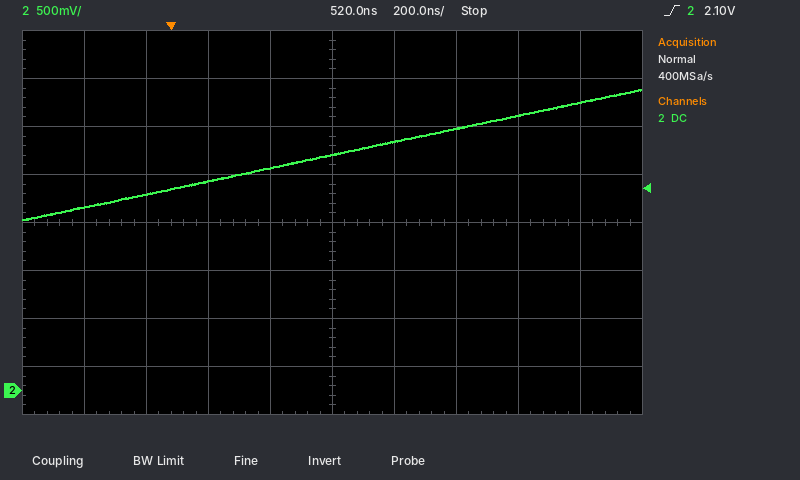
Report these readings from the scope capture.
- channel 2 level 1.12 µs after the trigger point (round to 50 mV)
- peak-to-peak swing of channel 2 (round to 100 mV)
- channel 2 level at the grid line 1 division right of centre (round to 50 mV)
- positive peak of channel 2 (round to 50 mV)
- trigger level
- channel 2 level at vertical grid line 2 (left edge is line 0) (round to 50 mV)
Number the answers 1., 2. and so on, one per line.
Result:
1. 2.85 V
2. 1.40 V
3. 2.60 V
4. 3.15 V
5. 2.10 V
6. 2.05 V
